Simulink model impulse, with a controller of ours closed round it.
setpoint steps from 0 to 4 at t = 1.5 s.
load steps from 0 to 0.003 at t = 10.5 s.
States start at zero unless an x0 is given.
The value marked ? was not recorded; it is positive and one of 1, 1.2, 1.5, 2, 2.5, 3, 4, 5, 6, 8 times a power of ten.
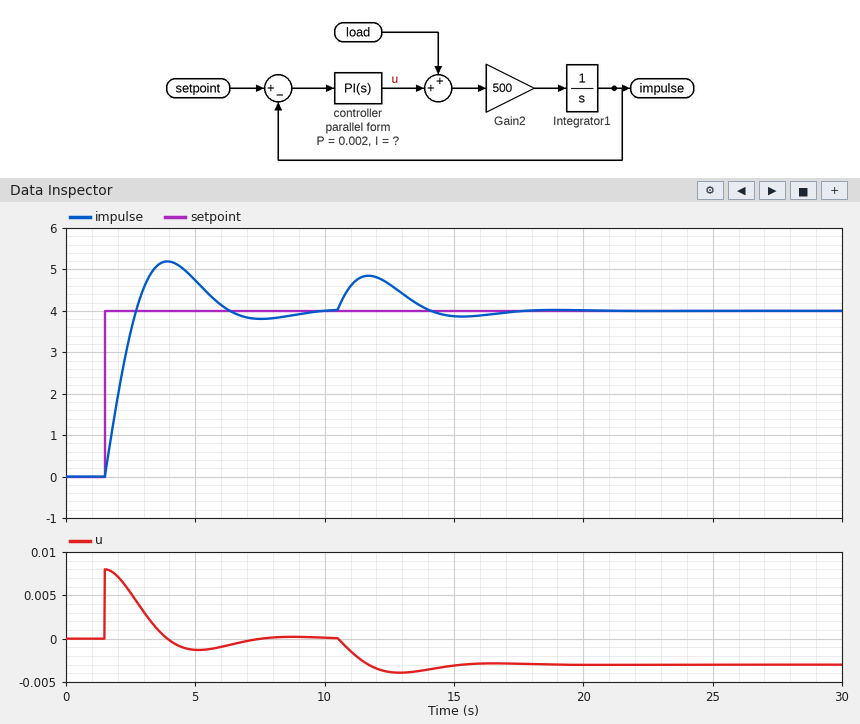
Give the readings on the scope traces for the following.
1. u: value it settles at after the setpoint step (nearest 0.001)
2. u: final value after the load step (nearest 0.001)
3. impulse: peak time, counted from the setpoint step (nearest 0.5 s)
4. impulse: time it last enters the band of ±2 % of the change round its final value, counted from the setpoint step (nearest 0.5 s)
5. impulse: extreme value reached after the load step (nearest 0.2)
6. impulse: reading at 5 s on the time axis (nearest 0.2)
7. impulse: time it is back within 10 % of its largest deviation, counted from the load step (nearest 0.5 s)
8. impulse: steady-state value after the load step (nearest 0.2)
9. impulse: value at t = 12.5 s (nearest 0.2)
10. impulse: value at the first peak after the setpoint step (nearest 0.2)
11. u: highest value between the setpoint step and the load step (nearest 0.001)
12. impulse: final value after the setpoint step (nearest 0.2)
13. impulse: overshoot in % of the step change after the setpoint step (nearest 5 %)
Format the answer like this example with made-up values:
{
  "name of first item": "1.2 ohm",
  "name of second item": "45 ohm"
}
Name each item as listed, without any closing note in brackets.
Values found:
{
  "u: value it settles at after the setpoint step": "0.000",
  "u: final value after the load step": "-0.003",
  "impulse: peak time, counted from the setpoint step": "2.5 s",
  "impulse: time it last enters the band of ±2 % of the change round its final value, counted from the setpoint step": "7.5 s",
  "impulse: extreme value reached after the load step": "4.8",
  "impulse: reading at 5 s on the time axis": "4.8",
  "impulse: time it is back within 10 % of its largest deviation, counted from the load step": "6.0 s",
  "impulse: steady-state value after the load step": "4.0",
  "impulse: value at t = 12.5 s": "4.6",
  "impulse: value at the first peak after the setpoint step": "5.2",
  "u: highest value between the setpoint step and the load step": "0.008",
  "impulse: final value after the setpoint step": "4.0",
  "impulse: overshoot in % of the step change after the setpoint step": "30 %"
}
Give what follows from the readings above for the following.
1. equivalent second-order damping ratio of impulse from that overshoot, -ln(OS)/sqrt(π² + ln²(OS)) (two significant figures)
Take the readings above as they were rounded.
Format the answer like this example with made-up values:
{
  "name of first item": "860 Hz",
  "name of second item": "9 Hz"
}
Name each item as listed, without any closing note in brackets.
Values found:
{
  "equivalent second-order damping ratio of impulse from that overshoot, -ln(OS)/sqrt(π² + ln²(OS))": "0.36"
}
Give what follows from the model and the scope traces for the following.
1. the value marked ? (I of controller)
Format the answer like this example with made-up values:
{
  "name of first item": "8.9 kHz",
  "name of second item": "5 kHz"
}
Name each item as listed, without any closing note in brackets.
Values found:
{
  "the value marked ?": "0.002"
}
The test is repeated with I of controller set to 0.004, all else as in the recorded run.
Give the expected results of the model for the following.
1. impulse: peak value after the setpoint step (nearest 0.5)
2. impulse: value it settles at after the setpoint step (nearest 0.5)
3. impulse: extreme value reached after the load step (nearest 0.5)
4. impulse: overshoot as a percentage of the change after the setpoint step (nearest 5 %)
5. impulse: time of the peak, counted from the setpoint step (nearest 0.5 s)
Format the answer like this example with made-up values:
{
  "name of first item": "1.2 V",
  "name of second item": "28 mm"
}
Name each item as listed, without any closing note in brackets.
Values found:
{
  "impulse: peak value after the setpoint step": "5.5",
  "impulse: value it settles at after the setpoint step": "4.0",
  "impulse: extreme value reached after the load step": "4.5",
  "impulse: overshoot as a percentage of the change after the setpoint step": "40 %",
  "impulse: time of the peak, counted from the setpoint step": "2.0 s"
}
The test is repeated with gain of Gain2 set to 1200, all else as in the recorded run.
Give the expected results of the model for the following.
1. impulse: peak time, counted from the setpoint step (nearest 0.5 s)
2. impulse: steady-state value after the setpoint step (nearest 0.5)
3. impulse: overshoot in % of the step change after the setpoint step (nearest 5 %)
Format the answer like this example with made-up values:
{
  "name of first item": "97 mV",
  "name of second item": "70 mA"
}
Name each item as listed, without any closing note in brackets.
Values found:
{
  "impulse: peak time, counted from the setpoint step": "1.5 s",
  "impulse: steady-state value after the setpoint step": "4.0",
  "impulse: overshoot in % of the step change after the setpoint step": "20 %"
}
